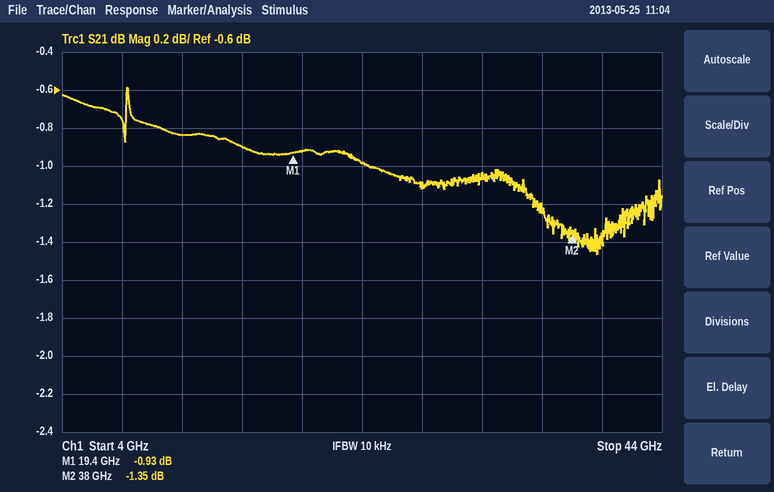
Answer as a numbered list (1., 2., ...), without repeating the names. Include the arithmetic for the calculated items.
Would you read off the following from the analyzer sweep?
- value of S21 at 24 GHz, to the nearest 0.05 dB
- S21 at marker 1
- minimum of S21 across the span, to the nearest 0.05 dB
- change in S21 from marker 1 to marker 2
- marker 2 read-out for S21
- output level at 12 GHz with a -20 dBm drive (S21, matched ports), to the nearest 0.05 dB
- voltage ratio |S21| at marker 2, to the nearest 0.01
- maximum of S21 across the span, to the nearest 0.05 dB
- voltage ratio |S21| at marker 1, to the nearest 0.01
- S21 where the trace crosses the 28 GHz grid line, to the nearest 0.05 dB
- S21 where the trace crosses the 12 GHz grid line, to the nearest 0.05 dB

1. -1.00 dB
2. -0.93 dB
3. -1.45 dB
4. -1.35 − (-0.93) = -0.42 dB
5. -1.35 dB
6. -20 dBm + (-0.85 dB) = -20.85 dBm
7. 10^(-1.35/20) ≈ 0.86
8. -0.60 dB
9. 10^(-0.93/20) ≈ 0.90
10. -1.10 dB
11. -0.85 dB
